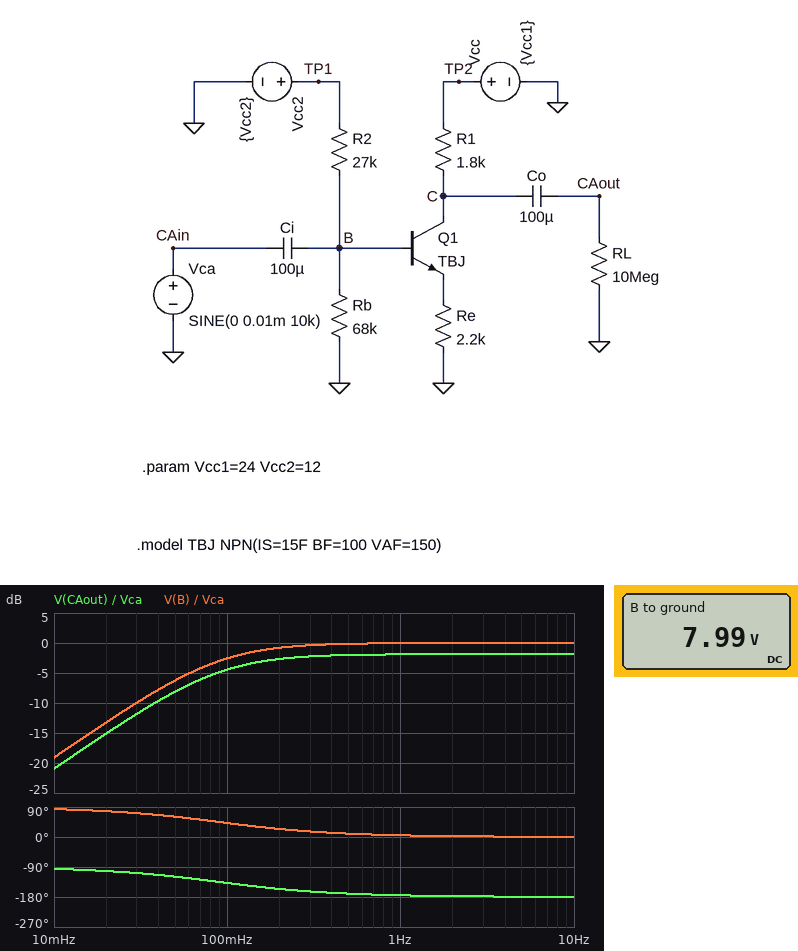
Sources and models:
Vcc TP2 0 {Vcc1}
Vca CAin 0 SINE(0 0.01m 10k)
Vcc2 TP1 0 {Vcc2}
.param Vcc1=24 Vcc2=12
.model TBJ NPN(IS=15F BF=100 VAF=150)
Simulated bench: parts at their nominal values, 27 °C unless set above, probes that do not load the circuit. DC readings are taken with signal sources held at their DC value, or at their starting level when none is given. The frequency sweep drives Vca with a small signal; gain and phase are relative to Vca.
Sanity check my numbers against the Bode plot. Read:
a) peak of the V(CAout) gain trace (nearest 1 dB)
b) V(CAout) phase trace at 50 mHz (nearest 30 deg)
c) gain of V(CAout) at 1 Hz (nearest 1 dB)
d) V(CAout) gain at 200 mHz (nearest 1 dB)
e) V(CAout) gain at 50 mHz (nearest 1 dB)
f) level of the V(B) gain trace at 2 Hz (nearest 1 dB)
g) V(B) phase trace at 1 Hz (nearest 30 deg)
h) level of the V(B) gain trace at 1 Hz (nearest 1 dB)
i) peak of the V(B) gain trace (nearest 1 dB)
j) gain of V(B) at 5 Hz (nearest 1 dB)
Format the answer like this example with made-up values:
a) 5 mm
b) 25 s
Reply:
a) -2 dB
b) -120 deg
c) -2 dB
d) -3 dB
e) -8 dB
f) 0 dB
g) 0 deg
h) 0 dB
i) 0 dB
j) 0 dB
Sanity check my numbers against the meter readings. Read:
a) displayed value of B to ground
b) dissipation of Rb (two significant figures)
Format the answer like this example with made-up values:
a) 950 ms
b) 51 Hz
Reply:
a) 7.99 V
b) 940 µW
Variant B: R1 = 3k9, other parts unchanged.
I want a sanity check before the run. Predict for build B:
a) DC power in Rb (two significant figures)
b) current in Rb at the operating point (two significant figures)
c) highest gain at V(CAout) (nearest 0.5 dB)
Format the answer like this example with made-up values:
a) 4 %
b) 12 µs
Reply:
a) 930 µW
b) 120 µA
c) 5.0 dB
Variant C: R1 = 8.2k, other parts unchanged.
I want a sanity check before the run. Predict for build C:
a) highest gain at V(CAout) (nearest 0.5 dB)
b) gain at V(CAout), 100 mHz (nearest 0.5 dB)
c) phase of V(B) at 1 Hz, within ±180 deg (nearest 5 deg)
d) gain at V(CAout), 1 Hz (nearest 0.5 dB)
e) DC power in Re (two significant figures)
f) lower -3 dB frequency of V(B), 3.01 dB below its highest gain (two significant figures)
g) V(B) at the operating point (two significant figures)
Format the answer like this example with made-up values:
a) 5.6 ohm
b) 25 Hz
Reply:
a) -1.0 dB
b) -21.0 dB
c) 45 deg
d) -4.0 dB
e) 13 mW
f) 970 mHz
g) 6.0 V
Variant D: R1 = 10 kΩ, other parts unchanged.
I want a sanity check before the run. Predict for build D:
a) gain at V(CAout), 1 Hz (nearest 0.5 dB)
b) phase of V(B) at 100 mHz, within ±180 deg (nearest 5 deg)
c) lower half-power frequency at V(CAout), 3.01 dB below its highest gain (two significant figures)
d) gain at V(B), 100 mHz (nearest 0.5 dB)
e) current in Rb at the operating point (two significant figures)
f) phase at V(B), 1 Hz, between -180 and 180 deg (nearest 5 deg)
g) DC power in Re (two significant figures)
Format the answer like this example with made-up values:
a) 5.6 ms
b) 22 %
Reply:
a) -3.5 dB
b) 85 deg
c) 940 mHz
d) -19.5 dB
e) 78 µA
f) 45 deg
g) 9.7 mW
